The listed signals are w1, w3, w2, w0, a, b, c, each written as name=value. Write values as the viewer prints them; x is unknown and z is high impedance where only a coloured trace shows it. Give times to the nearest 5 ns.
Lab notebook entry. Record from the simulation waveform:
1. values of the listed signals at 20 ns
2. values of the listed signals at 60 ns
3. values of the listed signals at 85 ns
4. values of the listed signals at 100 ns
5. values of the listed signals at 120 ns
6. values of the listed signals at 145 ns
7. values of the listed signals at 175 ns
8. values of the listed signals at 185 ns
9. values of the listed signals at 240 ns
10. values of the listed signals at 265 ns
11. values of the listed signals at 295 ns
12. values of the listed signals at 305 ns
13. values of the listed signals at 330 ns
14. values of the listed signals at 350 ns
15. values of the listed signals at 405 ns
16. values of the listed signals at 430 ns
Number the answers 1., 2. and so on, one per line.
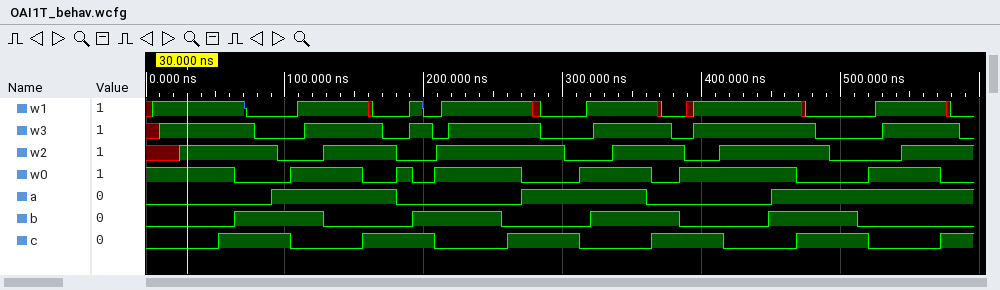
1. w1=1, w3=1, w2=x, w0=1, a=0, b=0, c=0
2. w1=1, w3=1, w2=1, w0=1, a=0, b=0, c=1
3. w1=0, w3=0, w2=1, w0=0, a=0, b=1, c=1
4. w1=0, w3=0, w2=0, w0=0, a=1, b=1, c=1
5. w1=1, w3=1, w2=0, w0=1, a=1, b=1, c=0
6. w1=1, w3=1, w2=1, w0=1, a=1, b=0, c=0
7. w1=0, w3=0, w2=1, w0=0, a=1, b=0, c=1
8. w1=0, w3=0, w2=0, w0=1, a=0, b=0, c=1
9. w1=1, w3=1, w2=1, w0=1, a=0, b=1, c=0
10. w1=1, w3=1, w2=1, w0=1, a=0, b=0, c=1
11. w1=0, w3=0, w2=1, w0=0, a=1, b=0, c=1
12. w1=0, w3=0, w2=0, w0=0, a=1, b=0, c=1
13. w1=1, w3=1, w2=0, w0=1, a=1, b=1, c=0
14. w1=1, w3=1, w2=1, w0=1, a=1, b=1, c=0
15. w1=1, w3=1, w2=0, w0=1, a=0, b=0, c=1
16. w1=1, w3=1, w2=1, w0=1, a=0, b=0, c=0
